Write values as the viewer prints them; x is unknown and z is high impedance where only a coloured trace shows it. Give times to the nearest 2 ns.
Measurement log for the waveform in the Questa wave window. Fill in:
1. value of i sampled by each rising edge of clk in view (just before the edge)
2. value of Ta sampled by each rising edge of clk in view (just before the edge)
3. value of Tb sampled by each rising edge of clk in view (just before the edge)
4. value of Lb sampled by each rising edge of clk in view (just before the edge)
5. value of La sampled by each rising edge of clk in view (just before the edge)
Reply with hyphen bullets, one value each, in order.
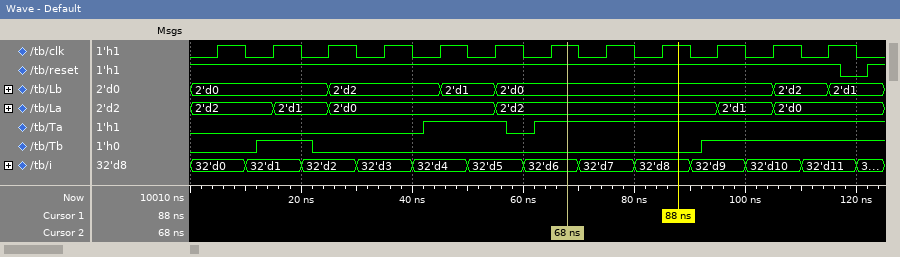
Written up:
- 32'd0, 32'd1, 32'd2, 32'd3, 32'd4, 32'd5, 32'd6, 32'd7, 32'd8, 32'd9, 32'd10, 32'd11
- 0 0 0 0 1 1 1 1 1 1 1 1
- 0 1 0 0 0 0 0 0 0 1 1 1
- 2'd0, 2'd0, 2'd0, 2'd2, 2'd2, 2'd1, 2'd0, 2'd0, 2'd0, 2'd0, 2'd0, 2'd2
- 2'd2, 2'd2, 2'd1, 2'd0, 2'd0, 2'd0, 2'd2, 2'd2, 2'd2, 2'd2, 2'd1, 2'd0
